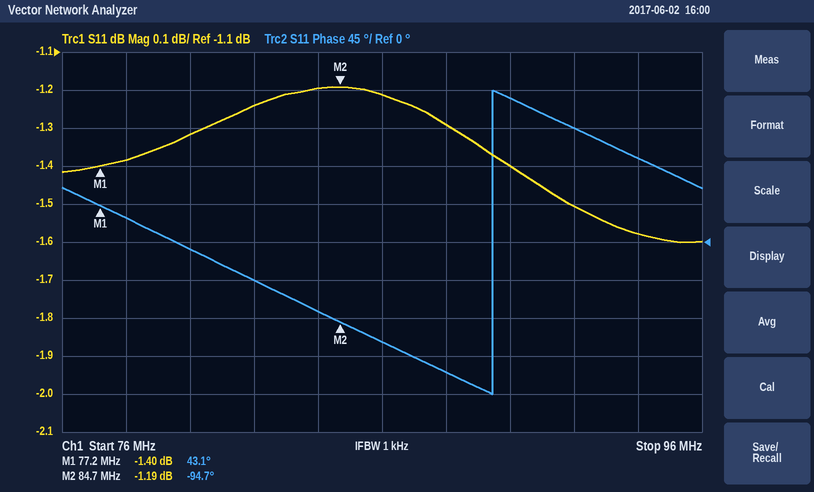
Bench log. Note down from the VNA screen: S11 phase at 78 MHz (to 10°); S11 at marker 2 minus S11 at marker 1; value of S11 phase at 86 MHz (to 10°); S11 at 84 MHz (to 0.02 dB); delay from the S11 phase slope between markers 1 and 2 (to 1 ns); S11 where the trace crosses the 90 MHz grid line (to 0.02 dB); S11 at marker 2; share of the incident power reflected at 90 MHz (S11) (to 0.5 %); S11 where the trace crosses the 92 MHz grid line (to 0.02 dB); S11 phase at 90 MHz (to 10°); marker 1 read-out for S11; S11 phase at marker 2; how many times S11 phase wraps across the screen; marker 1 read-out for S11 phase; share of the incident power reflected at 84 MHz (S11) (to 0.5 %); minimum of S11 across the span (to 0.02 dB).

30°
0.21 dB
-120°
-1.20 dB
51 ns
-1.40 dB
-1.19 dB
72.5 %
-1.50 dB
170°
-1.40 dB
-94.7°
1
43.1°
76.0 %
-1.60 dB
